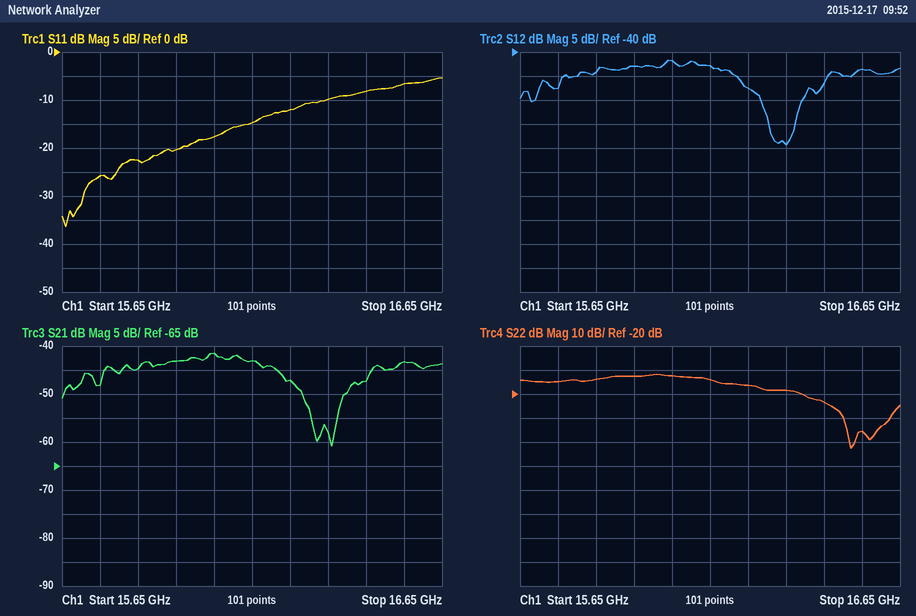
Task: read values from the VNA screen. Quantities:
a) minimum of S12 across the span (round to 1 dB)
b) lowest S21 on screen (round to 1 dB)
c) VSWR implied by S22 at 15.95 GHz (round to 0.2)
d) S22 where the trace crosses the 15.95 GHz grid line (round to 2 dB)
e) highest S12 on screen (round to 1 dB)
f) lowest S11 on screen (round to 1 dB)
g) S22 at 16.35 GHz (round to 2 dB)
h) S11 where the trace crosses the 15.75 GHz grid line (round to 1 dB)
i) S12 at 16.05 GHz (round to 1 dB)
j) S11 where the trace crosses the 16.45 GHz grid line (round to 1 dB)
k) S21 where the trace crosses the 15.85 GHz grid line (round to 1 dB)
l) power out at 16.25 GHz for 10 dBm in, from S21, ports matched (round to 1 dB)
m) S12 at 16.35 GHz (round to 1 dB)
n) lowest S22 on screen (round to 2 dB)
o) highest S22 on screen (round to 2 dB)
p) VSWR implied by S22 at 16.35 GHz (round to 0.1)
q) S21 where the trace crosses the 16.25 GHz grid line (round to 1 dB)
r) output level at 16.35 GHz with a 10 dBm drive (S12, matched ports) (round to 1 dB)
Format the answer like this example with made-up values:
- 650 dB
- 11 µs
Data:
- -59 dB
- -61 dB
- 1.6
- -12 dB
- -42 dB
- -36 dB
- -18 dB
- -26 dB
- -42 dB
- -8 dB
- -45 dB
- -37 dBm
- -59 dB
- -42 dB
- -12 dB
- 1.3
- -47 dB
- -49 dBm
